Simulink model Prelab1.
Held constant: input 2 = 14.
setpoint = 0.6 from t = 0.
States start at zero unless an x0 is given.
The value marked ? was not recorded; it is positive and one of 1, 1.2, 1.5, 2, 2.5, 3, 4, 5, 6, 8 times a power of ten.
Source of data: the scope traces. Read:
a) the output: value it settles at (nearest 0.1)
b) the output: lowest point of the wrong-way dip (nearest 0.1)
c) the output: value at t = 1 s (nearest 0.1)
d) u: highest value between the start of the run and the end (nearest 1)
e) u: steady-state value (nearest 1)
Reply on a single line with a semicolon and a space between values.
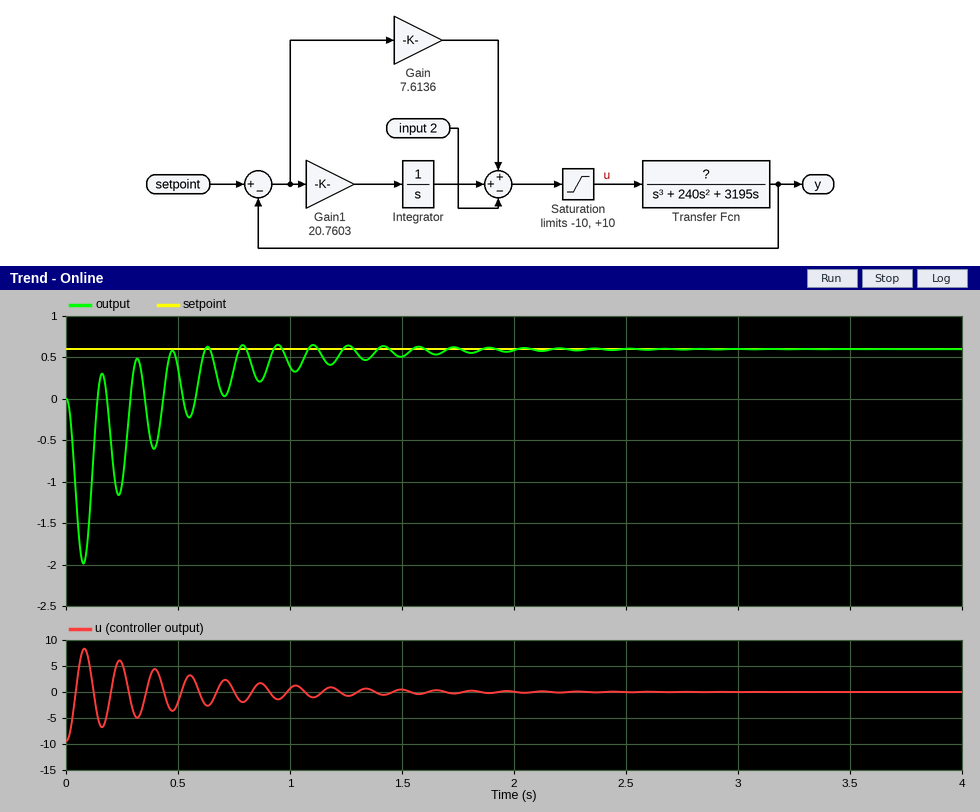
0.6; -2.0; 0.4; 8; 0
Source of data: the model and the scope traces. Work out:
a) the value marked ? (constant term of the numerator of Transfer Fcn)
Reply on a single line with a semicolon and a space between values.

50000
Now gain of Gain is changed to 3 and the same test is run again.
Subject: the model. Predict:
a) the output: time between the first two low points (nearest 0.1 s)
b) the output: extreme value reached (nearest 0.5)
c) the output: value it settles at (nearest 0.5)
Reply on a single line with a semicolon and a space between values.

0.3 s; -5.0; 0.5
